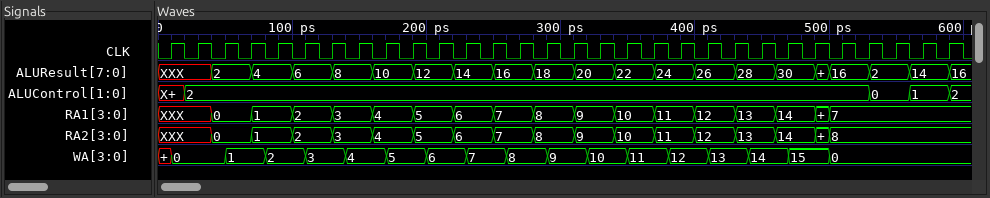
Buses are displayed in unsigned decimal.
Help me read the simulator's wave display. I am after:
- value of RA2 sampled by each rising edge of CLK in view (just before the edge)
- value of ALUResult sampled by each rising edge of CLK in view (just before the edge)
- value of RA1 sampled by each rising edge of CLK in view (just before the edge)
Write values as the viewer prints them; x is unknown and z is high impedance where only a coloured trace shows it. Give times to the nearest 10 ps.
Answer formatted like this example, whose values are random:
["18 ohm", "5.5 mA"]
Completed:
["XXX, XXX, 0, 0, 1, 2, 2, 3, 4, 4, 5, 6, 6, 7, 8, 8, 9, 10, 10, 11, 12, 12, 13, 14, 14, 8, 8, 8, 8, 8", "XXX, XXX, 2, 2, 4, 6, 6, 8, 10, 10, 12, 14, 14, 16, 18, 18, 20, 22, 22, 24, 26, 26, 28, 30, 30, 16, 16, 2, 14, 14", "XXX, XXX, 0, 0, 1, 2, 2, 3, 4, 4, 5, 6, 6, 7, 8, 8, 9, 10, 10, 11, 12, 12, 13, 14, 14, 7, 7, 7, 7, 7"]
